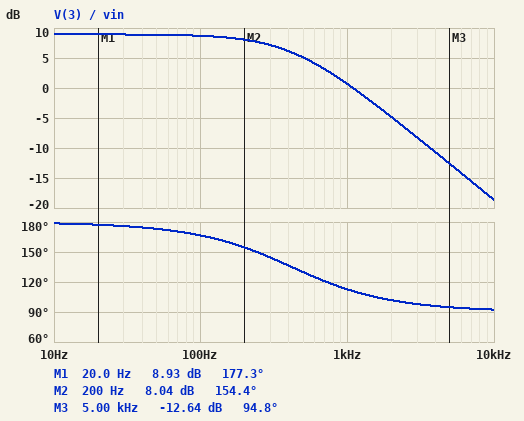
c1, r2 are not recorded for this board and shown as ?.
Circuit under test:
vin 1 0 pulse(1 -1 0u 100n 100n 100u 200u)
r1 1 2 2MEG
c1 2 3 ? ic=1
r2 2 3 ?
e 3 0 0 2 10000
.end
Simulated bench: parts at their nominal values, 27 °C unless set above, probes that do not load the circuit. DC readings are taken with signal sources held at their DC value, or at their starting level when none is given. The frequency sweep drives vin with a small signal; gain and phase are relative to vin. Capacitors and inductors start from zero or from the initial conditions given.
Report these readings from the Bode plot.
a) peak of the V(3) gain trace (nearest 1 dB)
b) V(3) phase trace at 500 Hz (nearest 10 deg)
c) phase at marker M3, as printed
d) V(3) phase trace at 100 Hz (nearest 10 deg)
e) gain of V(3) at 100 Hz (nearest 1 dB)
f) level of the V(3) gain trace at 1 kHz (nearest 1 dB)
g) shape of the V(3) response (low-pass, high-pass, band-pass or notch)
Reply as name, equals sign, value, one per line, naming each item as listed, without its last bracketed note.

peak of the V(3) gain trace = 9 dB
V(3) phase trace at 500 Hz = 130 deg
phase at marker M3, as printed = 94.8 deg
V(3) phase trace at 100 Hz = 170 deg
gain of V(3) at 100 Hz = 9 dB
level of the V(3) gain trace at 1 kHz = 1 dB
shape of the V(3) response = low-pass
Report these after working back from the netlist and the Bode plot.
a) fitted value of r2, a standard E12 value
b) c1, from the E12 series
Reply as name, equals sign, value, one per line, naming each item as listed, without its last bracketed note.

fitted value of r2, a standard E12 value = 5.6 MΩ
c1, from the E12 series = 68 pF
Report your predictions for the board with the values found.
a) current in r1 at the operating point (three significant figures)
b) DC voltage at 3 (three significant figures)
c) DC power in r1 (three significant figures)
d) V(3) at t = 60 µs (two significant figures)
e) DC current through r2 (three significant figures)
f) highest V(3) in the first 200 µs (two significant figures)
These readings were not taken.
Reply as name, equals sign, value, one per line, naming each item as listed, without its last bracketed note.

current in r1 at the operating point = 500 nA
DC voltage at 3 = -2.80 V
DC power in r1 = 500 nW
V(3) at t = 60 µs = -450 mV
DC current through r2 = 500 nA
highest V(3) in the first 200 µs = -120 mV
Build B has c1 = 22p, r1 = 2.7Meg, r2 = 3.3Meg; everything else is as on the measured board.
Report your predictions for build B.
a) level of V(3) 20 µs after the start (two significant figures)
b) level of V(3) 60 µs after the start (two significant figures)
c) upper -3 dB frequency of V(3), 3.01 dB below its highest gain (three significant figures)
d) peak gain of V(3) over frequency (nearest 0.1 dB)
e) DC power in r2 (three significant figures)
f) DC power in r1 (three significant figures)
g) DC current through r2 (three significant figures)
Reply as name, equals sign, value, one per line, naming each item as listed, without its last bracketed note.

level of V(3) 20 µs after the start = -470 mV
level of V(3) 60 µs after the start = 250 mV
upper -3 dB frequency of V(3), 3.01 dB below its highest gain = 2.19 kHz
peak gain of V(3) over frequency = 1.7 dB
DC power in r2 = 453 nW
DC power in r1 = 370 nW
DC current through r2 = 370 nA
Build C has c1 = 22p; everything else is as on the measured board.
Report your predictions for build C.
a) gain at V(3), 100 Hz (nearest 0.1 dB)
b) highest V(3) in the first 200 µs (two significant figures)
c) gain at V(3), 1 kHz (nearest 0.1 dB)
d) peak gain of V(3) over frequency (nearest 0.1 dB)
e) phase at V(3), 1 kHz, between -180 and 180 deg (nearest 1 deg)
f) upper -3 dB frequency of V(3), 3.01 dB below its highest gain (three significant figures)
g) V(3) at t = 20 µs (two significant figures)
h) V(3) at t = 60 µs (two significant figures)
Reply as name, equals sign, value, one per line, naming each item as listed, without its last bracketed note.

gain at V(3), 100 Hz = 8.9 dB
highest V(3) in the first 200 µs = 1.1 V
gain at V(3), 1 kHz = 6.9 dB
peak gain of V(3) over frequency = 8.9 dB
phase at V(3), 1 kHz, between -180 and 180 deg = 142 deg
upper -3 dB frequency of V(3), 3.01 dB below its highest gain = 1.29 kHz
V(3) at t = 20 µs = -430 mV
V(3) at t = 60 µs = 460 mV
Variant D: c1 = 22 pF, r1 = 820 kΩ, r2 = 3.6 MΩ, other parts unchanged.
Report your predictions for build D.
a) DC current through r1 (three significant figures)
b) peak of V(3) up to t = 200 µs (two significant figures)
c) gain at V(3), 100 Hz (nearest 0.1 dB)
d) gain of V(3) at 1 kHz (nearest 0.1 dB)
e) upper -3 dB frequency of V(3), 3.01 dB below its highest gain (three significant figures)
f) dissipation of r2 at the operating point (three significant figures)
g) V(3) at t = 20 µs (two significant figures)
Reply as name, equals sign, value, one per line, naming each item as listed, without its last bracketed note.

DC current through r1 = 1.22 µA
peak of V(3) up to t = 200 µs = 2.9 V
gain at V(3), 100 Hz = 12.8 dB
gain of V(3) at 1 kHz = 11.9 dB
upper -3 dB frequency of V(3), 3.01 dB below its highest gain = 2.01 kHz
dissipation of r2 at the operating point = 5.35 µW
V(3) at t = 20 µs = 200 mV
